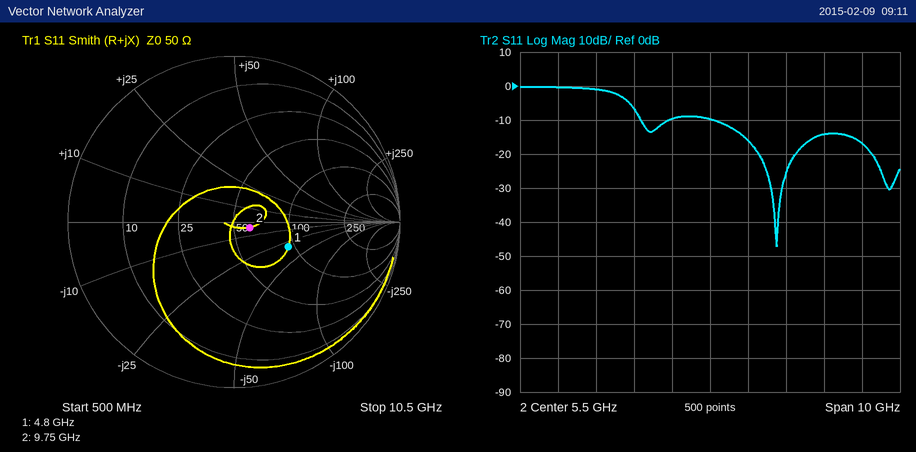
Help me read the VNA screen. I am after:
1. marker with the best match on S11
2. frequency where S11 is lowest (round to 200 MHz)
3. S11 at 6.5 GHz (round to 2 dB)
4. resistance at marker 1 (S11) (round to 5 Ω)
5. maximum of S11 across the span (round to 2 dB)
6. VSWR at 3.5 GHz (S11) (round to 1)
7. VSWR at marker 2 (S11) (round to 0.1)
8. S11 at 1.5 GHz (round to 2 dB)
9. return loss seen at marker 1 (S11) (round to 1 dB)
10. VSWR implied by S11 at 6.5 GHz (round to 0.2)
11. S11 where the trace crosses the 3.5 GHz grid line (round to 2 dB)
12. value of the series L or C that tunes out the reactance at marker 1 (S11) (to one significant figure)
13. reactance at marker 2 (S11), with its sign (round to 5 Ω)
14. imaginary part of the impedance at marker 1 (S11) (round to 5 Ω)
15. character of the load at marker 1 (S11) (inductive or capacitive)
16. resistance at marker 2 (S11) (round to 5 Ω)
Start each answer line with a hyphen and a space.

- marker 2
- 7.2 GHz
- -16 dB
- 90 Ω
- 0 dB
- 3
- 1.2
- 0 dB
- 9 dB
- 1.4
- -6 dB
- 1 nH
- -5 Ω
- -30 Ω
- capacitive
- 60 Ω
